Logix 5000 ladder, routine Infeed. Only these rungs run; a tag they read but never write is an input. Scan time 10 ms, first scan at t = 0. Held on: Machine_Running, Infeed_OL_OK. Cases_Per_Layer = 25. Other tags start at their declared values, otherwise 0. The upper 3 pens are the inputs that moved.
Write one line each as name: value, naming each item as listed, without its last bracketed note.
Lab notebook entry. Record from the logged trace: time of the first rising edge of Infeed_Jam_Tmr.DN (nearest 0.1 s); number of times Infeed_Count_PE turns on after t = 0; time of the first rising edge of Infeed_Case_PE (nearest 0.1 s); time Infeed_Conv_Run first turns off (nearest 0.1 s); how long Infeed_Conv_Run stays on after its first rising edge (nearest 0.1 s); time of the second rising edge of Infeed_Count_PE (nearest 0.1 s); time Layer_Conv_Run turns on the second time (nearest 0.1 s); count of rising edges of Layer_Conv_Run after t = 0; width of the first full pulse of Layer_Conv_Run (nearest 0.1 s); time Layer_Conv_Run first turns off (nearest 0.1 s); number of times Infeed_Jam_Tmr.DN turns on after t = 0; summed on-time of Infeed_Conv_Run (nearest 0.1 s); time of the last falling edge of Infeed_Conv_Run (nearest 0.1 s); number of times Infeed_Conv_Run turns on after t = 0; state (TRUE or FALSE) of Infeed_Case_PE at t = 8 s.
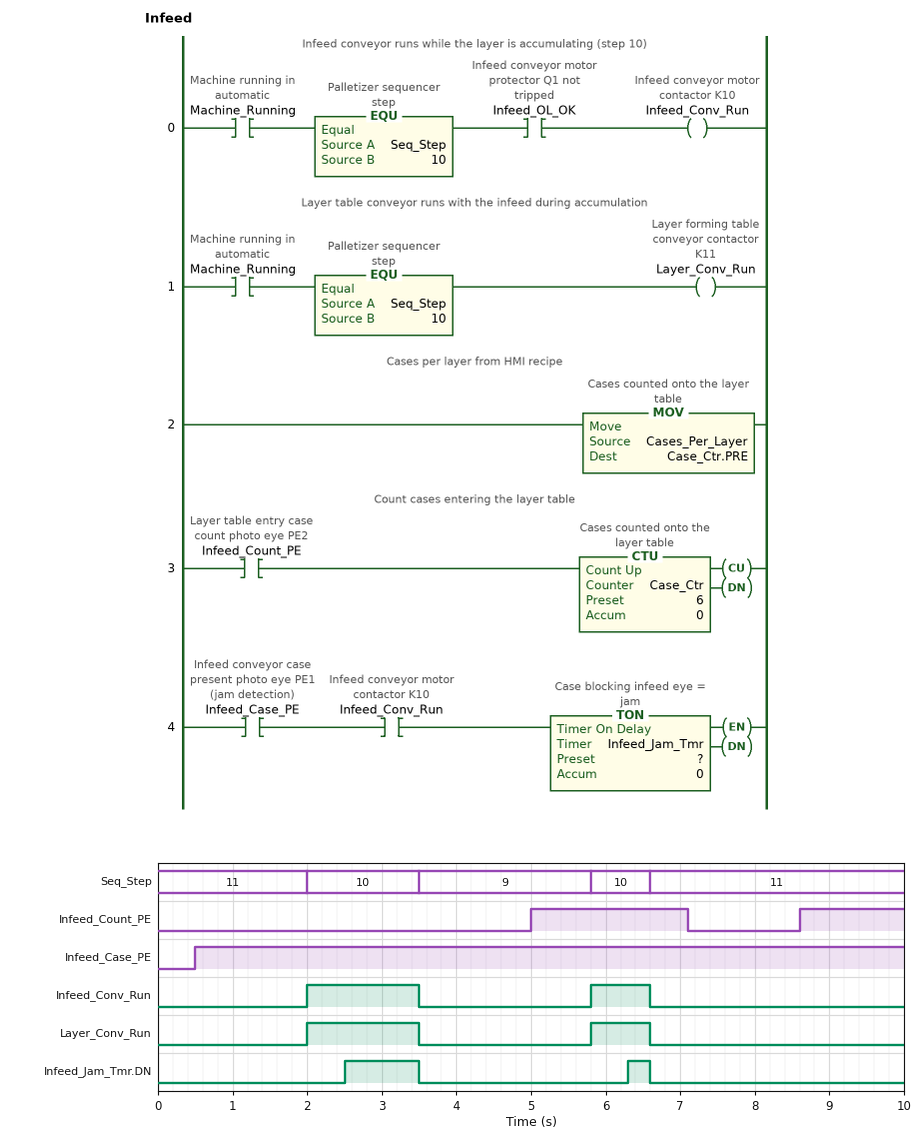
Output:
time of the first rising edge of Infeed_Jam_Tmr.DN: 2.5 s
number of times Infeed_Count_PE turns on after t = 0: 2
time of the first rising edge of Infeed_Case_PE: 0.5 s
time Infeed_Conv_Run first turns off: 3.5 s
how long Infeed_Conv_Run stays on after its first rising edge: 1.5 s
time of the second rising edge of Infeed_Count_PE: 8.6 s
time Layer_Conv_Run turns on the second time: 5.8 s
count of rising edges of Layer_Conv_Run after t = 0: 2
width of the first full pulse of Layer_Conv_Run: 1.5 s
time Layer_Conv_Run first turns off: 3.5 s
number of times Infeed_Jam_Tmr.DN turns on after t = 0: 2
summed on-time of Infeed_Conv_Run: 2.3 s
time of the last falling edge of Infeed_Conv_Run: 6.6 s
number of times Infeed_Conv_Run turns on after t = 0: 2
state (TRUE or FALSE) of Infeed_Case_PE at t = 8 s: TRUE
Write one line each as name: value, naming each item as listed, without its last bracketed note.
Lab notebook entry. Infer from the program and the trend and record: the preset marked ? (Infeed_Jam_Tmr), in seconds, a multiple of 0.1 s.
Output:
the preset marked ? (Infeed_Jam_Tmr), in seconds, a multiple of 0.1 s: 0.5 s
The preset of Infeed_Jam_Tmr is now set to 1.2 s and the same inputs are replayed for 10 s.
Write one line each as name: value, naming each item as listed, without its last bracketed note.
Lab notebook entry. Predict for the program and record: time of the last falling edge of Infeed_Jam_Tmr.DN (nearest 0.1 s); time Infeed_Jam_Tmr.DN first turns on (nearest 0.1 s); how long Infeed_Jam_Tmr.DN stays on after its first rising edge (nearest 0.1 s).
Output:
time of the last falling edge of Infeed_Jam_Tmr.DN: 3.5 s
time Infeed_Jam_Tmr.DN first turns on: 3.2 s
how long Infeed_Jam_Tmr.DN stays on after its first rising edge: 0.3 s
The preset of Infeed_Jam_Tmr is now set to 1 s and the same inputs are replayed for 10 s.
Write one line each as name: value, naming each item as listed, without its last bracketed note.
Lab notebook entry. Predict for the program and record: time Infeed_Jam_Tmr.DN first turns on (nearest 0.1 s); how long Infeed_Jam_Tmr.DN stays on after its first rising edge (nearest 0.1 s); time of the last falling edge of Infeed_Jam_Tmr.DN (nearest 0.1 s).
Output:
time Infeed_Jam_Tmr.DN first turns on: 3.0 s
how long Infeed_Jam_Tmr.DN stays on after its first rising edge: 0.5 s
time of the last falling edge of Infeed_Jam_Tmr.DN: 3.5 s
